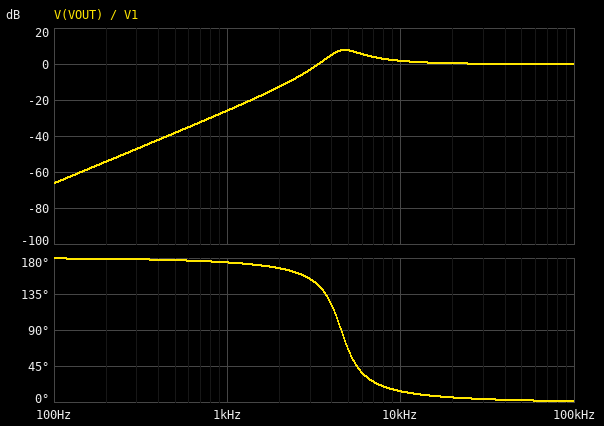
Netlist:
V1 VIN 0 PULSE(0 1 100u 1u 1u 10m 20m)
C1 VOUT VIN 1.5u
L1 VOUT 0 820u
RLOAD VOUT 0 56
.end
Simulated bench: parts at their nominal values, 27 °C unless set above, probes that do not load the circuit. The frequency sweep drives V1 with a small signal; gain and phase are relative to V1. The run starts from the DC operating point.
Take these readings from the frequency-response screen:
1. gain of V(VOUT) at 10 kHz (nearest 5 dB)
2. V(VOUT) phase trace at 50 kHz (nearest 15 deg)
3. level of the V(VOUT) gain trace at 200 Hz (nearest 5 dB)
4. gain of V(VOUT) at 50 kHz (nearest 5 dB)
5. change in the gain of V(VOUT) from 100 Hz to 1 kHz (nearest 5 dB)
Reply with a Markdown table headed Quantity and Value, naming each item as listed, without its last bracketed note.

| Quantity | Value |
|---|---|
| gain of V(VOUT) at 10 kHz | 0 dB |
| V(VOUT) phase trace at 50 kHz | 0 deg |
| level of the V(VOUT) gain trace at 200 Hz | -55 dB |
| gain of V(VOUT) at 50 kHz | 0 dB |
| change in the gain of V(VOUT) from 100 Hz to 1 kHz | 40 dB |
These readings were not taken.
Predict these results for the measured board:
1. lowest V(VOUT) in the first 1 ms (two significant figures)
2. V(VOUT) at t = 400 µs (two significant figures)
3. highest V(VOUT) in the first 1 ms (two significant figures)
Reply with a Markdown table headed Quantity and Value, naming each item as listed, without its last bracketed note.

| Quantity | Value |
|---|---|
| lowest V(VOUT) in the first 1 ms | -560 mV |
| V(VOUT) at t = 400 µs | -110 mV |
| highest V(VOUT) in the first 1 ms | 990 mV |
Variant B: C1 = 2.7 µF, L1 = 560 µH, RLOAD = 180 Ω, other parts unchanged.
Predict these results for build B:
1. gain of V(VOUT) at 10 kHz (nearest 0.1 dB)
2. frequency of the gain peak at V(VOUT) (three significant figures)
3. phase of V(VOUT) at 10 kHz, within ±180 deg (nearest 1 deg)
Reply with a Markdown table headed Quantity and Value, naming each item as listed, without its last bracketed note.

| Quantity | Value |
|---|---|
| gain of V(VOUT) at 10 kHz | 1.6 dB |
| frequency of the gain peak at V(VOUT) | 4.10 kHz |
| phase of V(VOUT) at 10 kHz, within ±180 deg | 2 deg |
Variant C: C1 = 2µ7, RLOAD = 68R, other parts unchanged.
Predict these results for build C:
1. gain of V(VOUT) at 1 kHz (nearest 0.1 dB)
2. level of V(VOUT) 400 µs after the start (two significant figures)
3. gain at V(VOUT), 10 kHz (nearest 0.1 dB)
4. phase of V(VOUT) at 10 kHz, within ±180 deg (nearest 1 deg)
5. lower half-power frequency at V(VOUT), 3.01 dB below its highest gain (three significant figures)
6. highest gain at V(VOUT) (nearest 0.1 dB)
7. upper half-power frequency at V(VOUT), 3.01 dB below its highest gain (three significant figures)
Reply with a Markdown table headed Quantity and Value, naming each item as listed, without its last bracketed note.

| Quantity | Value |
|---|---|
| gain of V(VOUT) at 1 kHz | -20.4 dB |
| level of V(VOUT) 400 µs after the start | 440 mV |
| gain at V(VOUT), 10 kHz | 1.0 dB |
| phase of V(VOUT) at 10 kHz, within ±180 deg | 6 deg |
| lower half-power frequency at V(VOUT), 3.01 dB below its highest gain | 3.06 kHz |
| highest gain at V(VOUT) | 11.9 dB |
| upper half-power frequency at V(VOUT), 3.01 dB below its highest gain | 4.01 kHz |
